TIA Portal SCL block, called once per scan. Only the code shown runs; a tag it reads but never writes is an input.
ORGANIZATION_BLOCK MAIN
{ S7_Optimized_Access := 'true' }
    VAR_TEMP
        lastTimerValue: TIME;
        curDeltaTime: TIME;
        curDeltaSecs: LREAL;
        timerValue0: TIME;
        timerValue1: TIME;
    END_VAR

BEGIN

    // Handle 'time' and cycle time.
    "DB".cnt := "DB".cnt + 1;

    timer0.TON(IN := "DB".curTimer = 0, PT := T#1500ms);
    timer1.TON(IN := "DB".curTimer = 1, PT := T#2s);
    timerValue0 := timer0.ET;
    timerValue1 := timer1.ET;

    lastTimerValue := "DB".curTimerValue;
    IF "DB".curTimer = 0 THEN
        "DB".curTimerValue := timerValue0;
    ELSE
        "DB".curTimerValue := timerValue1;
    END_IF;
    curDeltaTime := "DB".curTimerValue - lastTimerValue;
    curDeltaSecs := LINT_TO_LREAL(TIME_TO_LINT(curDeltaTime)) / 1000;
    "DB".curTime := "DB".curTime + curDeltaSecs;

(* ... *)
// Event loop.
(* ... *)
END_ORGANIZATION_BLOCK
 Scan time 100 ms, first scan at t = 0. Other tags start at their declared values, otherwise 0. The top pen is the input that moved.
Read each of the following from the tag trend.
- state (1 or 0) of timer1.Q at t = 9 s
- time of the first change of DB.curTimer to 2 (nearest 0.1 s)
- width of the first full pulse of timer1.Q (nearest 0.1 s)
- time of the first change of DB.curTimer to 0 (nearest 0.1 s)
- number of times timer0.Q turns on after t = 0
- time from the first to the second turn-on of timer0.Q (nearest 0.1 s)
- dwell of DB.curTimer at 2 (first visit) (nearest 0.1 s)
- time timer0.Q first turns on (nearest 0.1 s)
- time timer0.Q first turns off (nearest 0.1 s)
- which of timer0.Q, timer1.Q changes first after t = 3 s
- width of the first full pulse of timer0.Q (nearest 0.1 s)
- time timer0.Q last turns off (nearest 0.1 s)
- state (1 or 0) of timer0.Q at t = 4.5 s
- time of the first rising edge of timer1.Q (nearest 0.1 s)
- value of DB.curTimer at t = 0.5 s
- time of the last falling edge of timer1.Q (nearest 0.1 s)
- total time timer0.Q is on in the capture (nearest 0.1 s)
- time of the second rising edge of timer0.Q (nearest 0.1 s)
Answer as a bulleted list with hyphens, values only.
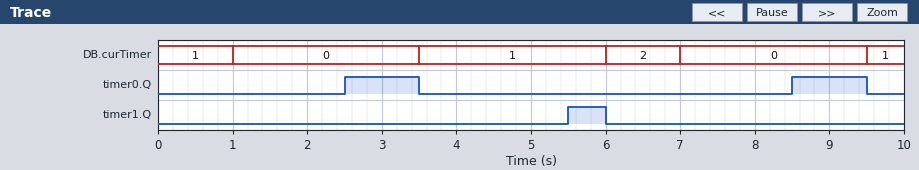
- 0
- 6.0 s
- 0.5 s
- 1.0 s
- 2
- 6.0 s
- 1.0 s
- 2.5 s
- 3.5 s
- timer0.Q
- 1.0 s
- 9.5 s
- 0
- 5.5 s
- 1
- 6.0 s
- 2.0 s
- 8.5 s
